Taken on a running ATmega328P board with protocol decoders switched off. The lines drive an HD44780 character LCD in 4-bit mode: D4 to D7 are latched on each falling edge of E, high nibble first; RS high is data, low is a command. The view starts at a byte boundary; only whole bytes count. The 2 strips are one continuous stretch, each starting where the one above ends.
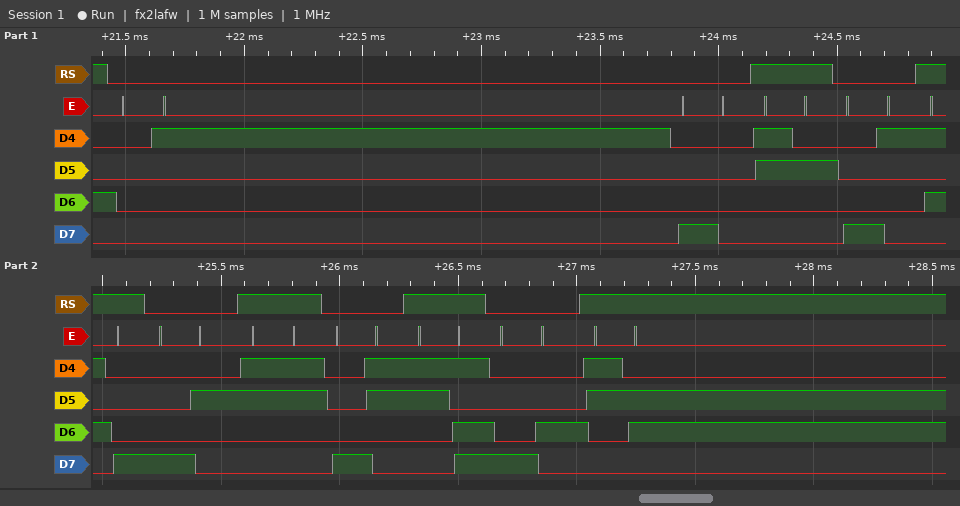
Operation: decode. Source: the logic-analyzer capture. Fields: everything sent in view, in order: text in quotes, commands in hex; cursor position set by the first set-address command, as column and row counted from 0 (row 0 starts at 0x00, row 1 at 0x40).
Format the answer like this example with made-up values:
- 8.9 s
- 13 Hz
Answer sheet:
- 0x01 0x80 "2" 0x81 "X" 0x82 "3" 0x83 "=" 0x84 "6"
- column 0, row 0
